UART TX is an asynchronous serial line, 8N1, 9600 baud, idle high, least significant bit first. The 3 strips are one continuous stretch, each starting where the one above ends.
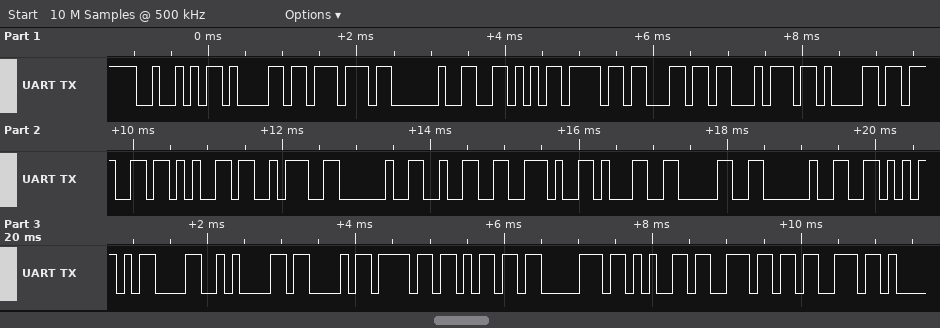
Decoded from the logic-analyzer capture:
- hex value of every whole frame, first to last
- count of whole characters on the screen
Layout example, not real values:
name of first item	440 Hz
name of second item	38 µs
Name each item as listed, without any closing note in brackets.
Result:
hex value of every whole frame, first to last	0x52 0x61 0x77 0x20 0x56 0x6F 0x6C 0x74 0x61 0x67 0x65 0x3A 0x20 0x32 0x2E 0x31 0x30 0x20 0x56 0x0D 0x0A 0x43 0x6F 0x6D 0x70 0x65 0x6E 0x73
count of whole characters on the screen	28
